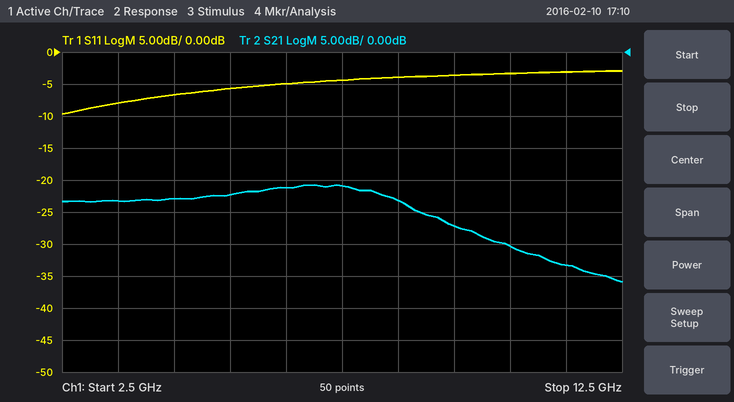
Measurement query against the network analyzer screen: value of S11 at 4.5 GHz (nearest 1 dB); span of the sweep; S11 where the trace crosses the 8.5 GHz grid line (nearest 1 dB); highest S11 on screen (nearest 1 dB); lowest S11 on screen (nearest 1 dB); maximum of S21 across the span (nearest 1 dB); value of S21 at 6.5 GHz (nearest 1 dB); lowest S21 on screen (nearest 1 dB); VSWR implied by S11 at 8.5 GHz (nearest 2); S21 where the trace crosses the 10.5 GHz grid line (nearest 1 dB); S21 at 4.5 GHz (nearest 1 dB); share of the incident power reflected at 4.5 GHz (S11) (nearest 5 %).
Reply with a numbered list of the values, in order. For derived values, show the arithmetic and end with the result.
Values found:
1. -7 dB
2. 10 GHz
3. -4 dB
4. -3 dB
5. -10 dB
6. -21 dB
7. -21 dB
8. -36 dB
9. |Γ| = 10^(-4/20) = 0.6310; VSWR = (1 + 0.6310)/(1 − 0.6310) ≈ 4
10. -30 dB
11. -23 dB
12. 10^(-7/10) ≈ 20 %
